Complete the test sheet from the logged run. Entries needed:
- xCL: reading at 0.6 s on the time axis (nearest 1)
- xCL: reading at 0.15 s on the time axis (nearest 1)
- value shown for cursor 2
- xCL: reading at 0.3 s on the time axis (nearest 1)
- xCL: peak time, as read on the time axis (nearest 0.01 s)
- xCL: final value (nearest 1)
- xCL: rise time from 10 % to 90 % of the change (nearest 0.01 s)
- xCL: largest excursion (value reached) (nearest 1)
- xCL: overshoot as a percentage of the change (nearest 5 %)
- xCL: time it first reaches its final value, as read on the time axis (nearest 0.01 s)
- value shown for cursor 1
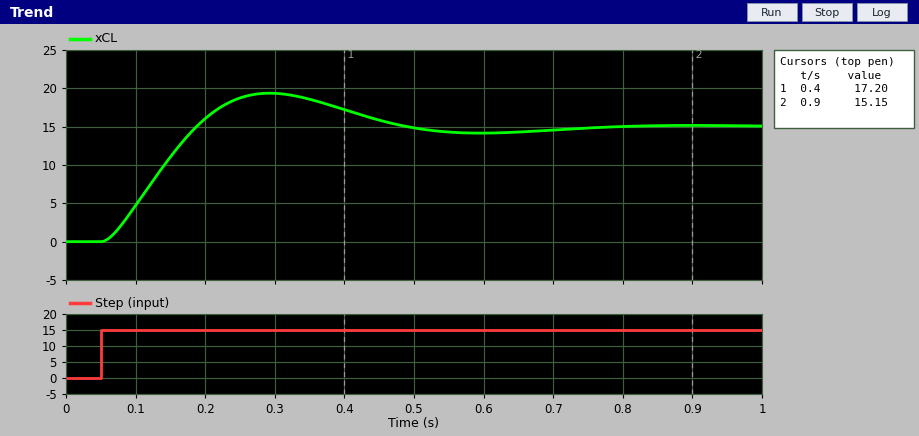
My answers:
14
11
15.15
19
0.29 s
15
0.10 s
19
30 %
0.19 s
17.20
